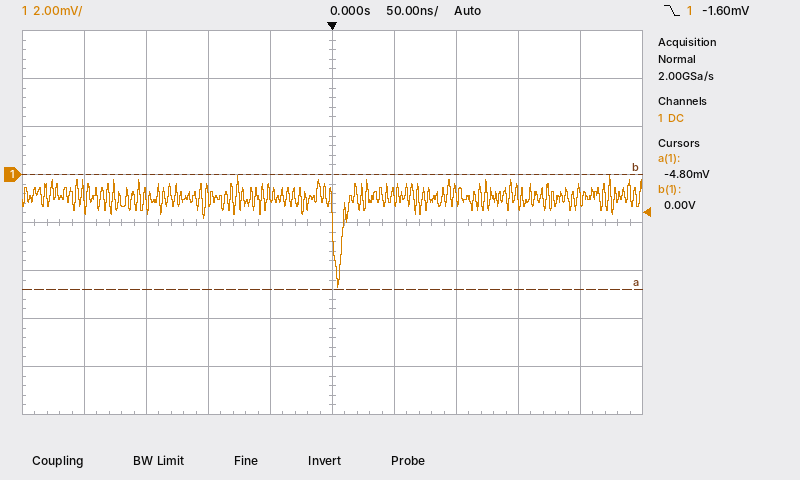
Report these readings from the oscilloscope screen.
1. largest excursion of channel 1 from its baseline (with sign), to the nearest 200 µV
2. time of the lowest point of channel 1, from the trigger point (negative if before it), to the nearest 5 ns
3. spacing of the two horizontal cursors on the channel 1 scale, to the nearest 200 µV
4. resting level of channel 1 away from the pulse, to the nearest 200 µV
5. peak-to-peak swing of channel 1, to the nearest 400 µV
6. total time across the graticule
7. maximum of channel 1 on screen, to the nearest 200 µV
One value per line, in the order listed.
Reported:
-3.8 mV
+5 ns
4.8 mV
-1.0 mV
4.8 mV
500 ns
0.0 mV
